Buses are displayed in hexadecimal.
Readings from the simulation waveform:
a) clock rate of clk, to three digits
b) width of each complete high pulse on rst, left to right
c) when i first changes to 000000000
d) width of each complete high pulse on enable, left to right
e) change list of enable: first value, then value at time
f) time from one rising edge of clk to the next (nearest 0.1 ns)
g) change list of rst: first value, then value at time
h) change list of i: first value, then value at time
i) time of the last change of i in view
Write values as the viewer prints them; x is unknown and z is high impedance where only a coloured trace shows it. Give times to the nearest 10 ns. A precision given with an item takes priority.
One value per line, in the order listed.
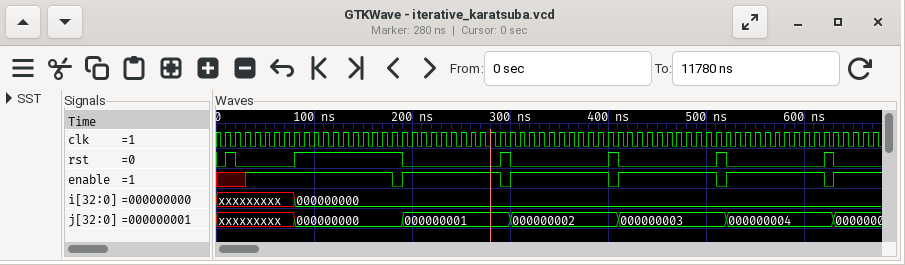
100 MHz
10 ns, 110 ns, 10 ns, 10 ns, 10 ns, 10 ns
80 ns
100 ns, 100 ns, 100 ns, 100 ns
x, 1 at 30 ns, 0 at 180 ns, 1 at 190 ns, 0 at 290 ns, 1 at 300 ns, 0 at 400 ns, 1 at 410 ns, 0 at 510 ns, 1 at 520 ns, 0 at 620 ns, 1 at 630 ns
10 ns
0, 1 at 10 ns, 0 at 20 ns, 1 at 80 ns, 0 at 190 ns, 1 at 290 ns, 0 at 300 ns, 1 at 400 ns, 0 at 410 ns, 1 at 510 ns, 0 at 520 ns, 1 at 620 ns, 0 at 630 ns
xxxxxxxxx, 000000000 at 80 ns
80 ns
